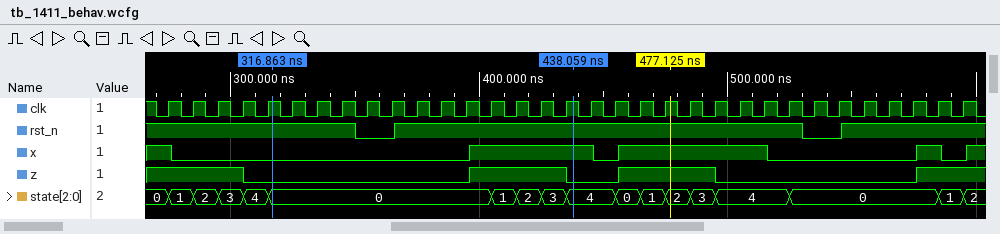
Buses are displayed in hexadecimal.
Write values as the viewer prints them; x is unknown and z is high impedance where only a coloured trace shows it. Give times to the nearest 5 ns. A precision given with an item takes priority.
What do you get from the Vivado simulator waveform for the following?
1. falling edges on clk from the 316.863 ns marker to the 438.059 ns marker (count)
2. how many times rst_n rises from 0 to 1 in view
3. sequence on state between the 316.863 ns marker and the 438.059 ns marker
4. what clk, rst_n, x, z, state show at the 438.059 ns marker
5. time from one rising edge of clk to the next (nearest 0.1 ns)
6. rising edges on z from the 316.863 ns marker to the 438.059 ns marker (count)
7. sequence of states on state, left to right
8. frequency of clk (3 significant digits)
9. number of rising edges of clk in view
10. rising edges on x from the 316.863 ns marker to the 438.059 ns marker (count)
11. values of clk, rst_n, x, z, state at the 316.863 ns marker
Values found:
12
2
0, 1, 2, 3, 4
clk=1, rst_n=1, x=1, z=0, state=4
10 ns
1
0, 1, 2, 3, 4, 0, 1, 2, 3, 4, 0, 1, 2, 3, 4, 0, 1, 2
100 MHz
33
1
clk=1, rst_n=1, x=0, z=0, state=0
